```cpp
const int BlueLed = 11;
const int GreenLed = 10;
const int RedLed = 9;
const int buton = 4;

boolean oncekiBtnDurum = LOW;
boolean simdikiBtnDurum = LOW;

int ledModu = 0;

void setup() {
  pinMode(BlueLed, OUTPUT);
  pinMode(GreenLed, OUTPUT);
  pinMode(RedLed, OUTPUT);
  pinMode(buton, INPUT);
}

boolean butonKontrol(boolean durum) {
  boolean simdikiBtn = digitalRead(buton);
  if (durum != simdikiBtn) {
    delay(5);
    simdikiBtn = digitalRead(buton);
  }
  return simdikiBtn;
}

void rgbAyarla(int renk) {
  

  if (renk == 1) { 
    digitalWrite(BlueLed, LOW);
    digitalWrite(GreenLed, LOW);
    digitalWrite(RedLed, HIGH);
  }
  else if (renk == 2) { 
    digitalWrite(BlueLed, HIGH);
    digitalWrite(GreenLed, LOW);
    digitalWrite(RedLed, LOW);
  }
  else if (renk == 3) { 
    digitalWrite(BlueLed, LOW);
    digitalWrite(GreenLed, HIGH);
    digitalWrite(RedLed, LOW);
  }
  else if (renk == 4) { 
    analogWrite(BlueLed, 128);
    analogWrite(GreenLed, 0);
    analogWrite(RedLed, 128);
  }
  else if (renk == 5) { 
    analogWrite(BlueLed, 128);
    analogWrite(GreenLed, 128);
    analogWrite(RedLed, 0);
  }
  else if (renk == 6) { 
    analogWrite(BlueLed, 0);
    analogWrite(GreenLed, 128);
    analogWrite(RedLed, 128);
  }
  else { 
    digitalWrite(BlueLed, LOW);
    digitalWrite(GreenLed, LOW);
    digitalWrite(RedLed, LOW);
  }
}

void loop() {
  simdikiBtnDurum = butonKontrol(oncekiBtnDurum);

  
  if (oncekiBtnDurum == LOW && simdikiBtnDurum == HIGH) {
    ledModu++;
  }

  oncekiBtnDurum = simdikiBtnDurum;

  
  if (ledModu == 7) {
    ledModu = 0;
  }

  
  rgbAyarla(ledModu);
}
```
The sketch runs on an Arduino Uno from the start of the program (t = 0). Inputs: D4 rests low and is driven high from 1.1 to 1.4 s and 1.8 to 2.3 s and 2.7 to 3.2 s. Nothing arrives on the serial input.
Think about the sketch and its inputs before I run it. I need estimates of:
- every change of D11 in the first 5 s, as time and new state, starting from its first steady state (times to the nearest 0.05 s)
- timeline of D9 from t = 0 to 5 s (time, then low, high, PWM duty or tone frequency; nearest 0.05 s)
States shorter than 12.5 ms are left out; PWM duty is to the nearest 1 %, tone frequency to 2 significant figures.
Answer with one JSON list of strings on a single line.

["0 s low; 1.8 s high; 2.7 s low", "0 s low; 1.1 s high; 1.8 s low"]
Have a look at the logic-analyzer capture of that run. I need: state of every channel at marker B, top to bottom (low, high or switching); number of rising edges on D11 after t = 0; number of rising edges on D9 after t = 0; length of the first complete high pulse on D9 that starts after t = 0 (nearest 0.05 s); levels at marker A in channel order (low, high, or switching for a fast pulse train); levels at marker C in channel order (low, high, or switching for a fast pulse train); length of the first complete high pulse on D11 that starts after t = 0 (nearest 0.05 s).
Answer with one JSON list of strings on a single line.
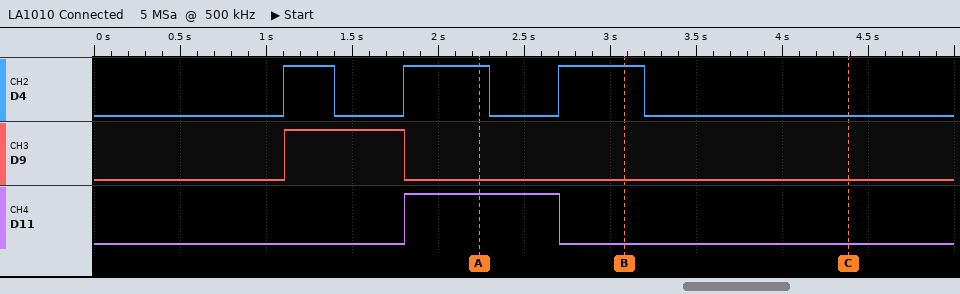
["D4 high, D9 low, D11 low", "1", "1", "0.70 s", "D4 high, D9 low, D11 high", "D4 low, D9 low, D11 low", "0.90 s"]
